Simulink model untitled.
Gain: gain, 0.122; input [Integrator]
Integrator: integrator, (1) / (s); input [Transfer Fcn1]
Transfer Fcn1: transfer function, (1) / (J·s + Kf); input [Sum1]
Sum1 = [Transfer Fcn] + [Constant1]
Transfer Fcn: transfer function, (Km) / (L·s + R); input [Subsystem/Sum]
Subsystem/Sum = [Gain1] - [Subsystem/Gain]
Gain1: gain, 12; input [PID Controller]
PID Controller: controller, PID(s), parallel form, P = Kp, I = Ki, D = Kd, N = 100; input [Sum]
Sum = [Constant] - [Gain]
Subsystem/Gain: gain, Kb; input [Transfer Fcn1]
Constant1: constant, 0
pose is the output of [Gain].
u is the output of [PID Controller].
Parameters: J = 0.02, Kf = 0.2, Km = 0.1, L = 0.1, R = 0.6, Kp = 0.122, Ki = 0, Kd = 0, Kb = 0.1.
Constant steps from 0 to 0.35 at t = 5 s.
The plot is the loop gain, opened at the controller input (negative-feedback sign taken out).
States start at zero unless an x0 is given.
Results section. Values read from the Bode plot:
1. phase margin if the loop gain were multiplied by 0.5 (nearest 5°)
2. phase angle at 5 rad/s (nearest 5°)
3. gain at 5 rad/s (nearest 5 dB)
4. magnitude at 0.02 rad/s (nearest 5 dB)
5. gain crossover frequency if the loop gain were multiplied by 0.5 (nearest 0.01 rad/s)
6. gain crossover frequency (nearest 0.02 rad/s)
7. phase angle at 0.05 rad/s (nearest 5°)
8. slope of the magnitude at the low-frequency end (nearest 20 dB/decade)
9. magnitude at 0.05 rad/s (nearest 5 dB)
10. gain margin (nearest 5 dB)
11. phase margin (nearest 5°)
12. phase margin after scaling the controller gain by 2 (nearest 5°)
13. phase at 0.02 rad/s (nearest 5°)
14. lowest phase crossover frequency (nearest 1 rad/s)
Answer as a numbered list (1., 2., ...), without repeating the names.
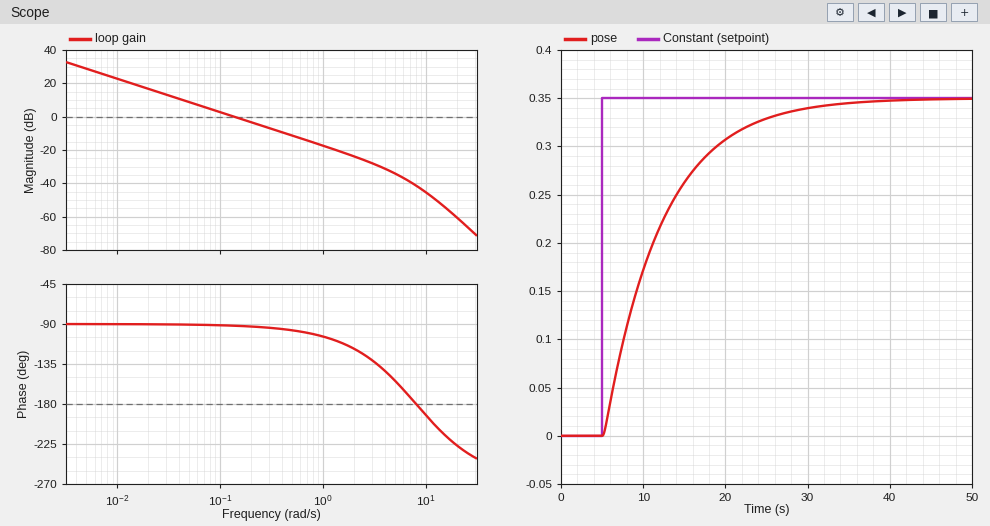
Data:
1. 90°
2. -155°
3. -35 dB
4. 15 dB
5. 0.07 rad/s
6. 0.14 rad/s
7. -90°
8. -20 dB/decade
9. 10 dB
10. 40 dB
11. 90°
12. 85°
13. -90°
14. 8 rad/s
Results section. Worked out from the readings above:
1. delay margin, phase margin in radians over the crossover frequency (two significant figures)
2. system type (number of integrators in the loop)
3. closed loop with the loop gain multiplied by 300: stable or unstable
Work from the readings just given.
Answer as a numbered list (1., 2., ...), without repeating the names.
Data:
1. 11 s
2. 1
3. unstable
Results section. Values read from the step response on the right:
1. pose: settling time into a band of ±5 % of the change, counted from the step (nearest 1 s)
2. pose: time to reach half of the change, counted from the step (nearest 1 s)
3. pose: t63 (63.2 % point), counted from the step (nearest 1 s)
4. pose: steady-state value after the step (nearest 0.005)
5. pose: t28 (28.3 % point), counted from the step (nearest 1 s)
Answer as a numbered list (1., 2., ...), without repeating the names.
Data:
1. 21 s
2. 5 s
3. 7 s
4. 0.350
5. 3 s
